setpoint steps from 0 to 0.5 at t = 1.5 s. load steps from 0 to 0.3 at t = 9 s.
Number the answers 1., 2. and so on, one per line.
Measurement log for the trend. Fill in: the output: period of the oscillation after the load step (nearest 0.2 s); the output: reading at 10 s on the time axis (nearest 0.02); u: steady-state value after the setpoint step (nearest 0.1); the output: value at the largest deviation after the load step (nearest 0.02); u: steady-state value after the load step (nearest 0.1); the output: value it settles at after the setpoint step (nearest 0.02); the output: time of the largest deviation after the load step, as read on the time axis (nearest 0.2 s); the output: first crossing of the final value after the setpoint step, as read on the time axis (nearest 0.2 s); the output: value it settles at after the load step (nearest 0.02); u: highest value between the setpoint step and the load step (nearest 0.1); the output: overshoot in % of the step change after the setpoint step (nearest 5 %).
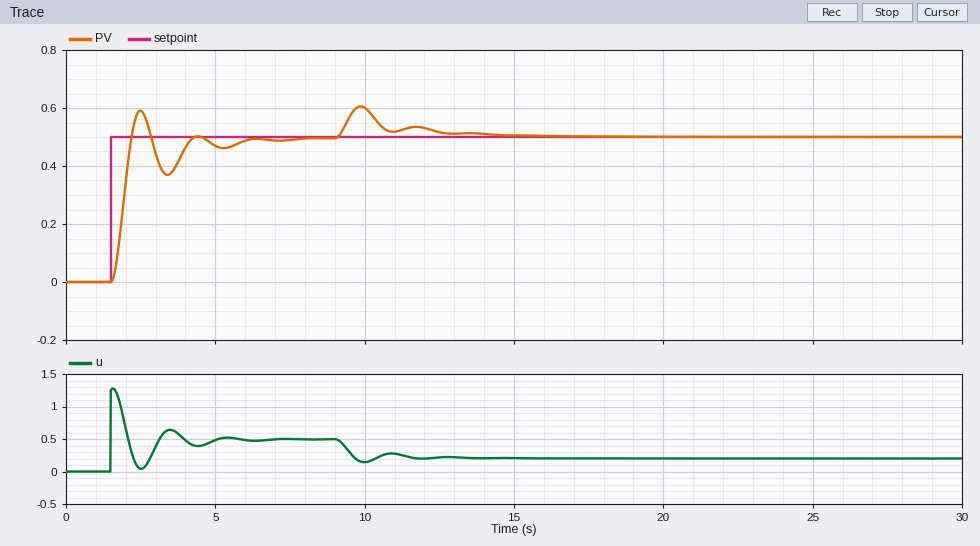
1. 1.8 s
2. 0.60
3. 0.5
4. 0.60
5. 0.2
6. 0.50
7. 9.8 s
8. 2.2 s
9. 0.50
10. 1.3
11. 20 %
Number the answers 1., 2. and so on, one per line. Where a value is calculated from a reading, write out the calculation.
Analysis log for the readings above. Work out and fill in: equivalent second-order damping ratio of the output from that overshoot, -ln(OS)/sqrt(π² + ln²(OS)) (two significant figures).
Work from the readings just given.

1. ln(0.2) = -1.609; 1.609 / sqrt(9.870 + 2.590) = 0.46
